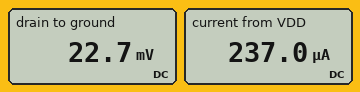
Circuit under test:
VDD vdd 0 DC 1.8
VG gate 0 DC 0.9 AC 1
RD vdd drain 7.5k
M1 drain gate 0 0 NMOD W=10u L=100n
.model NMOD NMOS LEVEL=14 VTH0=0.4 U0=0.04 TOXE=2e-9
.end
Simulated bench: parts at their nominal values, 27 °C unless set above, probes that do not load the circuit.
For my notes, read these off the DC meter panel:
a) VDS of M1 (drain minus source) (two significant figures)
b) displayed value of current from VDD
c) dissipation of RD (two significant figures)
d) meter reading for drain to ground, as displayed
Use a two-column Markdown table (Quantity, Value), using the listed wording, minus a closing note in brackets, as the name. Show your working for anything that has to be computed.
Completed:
| Quantity | Value |
|---|---|
| VDS of M1 (drain minus source) | 22.7 mV = 23 mV |
| displayed value of current from VDD | 237.0 µA |
| dissipation of RD | (1.8 V - 22.7 mV)^2 / 7.5 kΩ = 420 µW |
| meter reading for drain to ground, as displayed | 22.7 mV |
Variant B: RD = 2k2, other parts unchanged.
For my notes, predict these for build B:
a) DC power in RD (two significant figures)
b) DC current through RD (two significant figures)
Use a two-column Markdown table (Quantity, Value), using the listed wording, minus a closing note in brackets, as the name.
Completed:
| Quantity | Value |
|---|---|
| DC power in RD | 1.3 mW |
| DC current through RD | 780 µA |
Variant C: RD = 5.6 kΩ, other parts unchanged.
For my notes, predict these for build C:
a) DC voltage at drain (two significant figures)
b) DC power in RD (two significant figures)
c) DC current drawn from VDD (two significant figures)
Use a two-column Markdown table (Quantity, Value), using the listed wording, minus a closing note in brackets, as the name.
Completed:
| Quantity | Value |
|---|---|
| DC voltage at drain | 31 mV |
| DC power in RD | 560 µW |
| DC current drawn from VDD | 320 µA |
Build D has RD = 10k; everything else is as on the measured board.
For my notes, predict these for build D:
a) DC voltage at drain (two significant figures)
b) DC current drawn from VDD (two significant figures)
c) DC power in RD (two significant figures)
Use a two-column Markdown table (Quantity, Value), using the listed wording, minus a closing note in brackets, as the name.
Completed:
| Quantity | Value |
|---|---|
| DC voltage at drain | 17 mV |
| DC current drawn from VDD | 180 µA |
| DC power in RD | 320 µW |
